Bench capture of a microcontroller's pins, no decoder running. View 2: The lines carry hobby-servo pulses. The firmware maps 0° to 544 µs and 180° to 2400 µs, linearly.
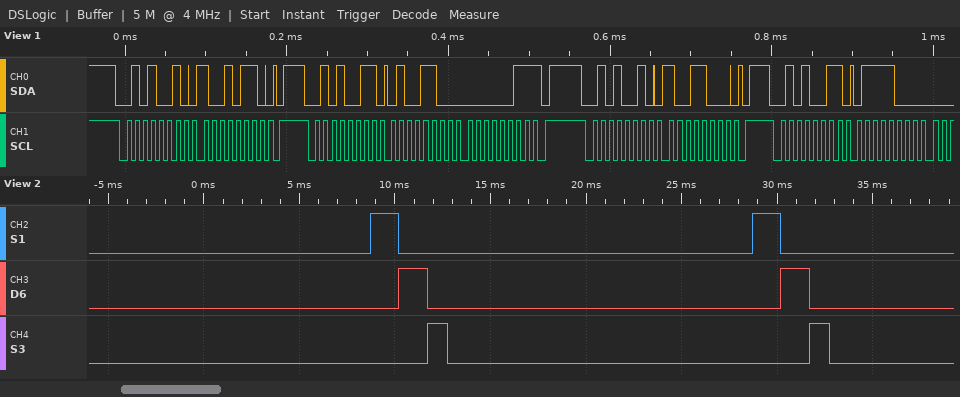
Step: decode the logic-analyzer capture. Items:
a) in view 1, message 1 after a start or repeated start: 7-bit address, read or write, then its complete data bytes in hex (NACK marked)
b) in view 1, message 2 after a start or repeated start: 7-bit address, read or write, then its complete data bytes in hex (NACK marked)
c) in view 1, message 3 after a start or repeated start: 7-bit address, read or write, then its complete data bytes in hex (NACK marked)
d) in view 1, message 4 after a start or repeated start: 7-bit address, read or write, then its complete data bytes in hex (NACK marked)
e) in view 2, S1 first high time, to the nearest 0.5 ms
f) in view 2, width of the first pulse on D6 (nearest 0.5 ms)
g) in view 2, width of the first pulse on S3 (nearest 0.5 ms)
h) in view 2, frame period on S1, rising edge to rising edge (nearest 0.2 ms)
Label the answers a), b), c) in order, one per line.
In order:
a) 0x29 write: 96
b) 0x29 read: 4C 03 NACK
c) 0x29 write: 98
d) 0x29 read: 78
e) 1.5 ms
f) 1.5 ms
g) 1.0 ms
h) 20.0 ms
